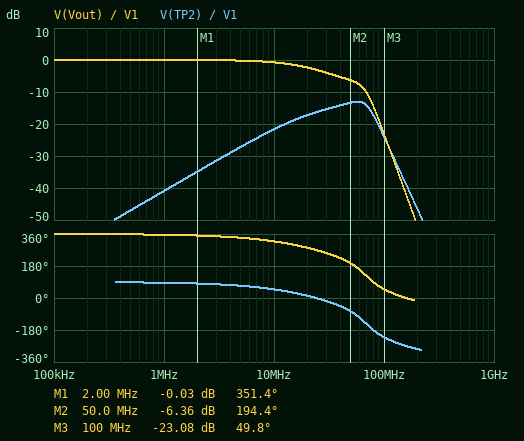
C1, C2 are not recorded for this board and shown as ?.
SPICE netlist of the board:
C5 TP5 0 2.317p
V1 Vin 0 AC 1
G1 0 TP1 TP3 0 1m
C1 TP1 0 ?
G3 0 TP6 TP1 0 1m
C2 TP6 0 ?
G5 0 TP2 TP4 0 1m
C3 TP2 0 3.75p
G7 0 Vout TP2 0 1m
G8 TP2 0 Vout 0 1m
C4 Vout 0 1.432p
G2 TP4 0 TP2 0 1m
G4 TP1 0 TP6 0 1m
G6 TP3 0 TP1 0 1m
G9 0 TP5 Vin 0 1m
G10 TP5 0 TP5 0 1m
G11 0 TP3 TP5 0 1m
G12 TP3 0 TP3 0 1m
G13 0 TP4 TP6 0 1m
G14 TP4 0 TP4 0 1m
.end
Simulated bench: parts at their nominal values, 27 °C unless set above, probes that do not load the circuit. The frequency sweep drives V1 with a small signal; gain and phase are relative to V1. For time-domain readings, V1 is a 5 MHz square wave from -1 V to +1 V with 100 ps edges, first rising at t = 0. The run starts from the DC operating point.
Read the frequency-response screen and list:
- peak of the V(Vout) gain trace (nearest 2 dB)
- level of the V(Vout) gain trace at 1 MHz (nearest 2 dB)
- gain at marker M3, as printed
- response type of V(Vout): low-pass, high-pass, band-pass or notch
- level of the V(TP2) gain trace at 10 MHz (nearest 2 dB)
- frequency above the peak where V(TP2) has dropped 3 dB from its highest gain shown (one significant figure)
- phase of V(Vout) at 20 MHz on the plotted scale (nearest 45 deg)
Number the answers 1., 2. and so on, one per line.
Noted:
1. 0 dB
2. 0 dB
3. -23.08 dB
4. low-pass
5. -22 dB
6. 80 MHz
7. 270 deg
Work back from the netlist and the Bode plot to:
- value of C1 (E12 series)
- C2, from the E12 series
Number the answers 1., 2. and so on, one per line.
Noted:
1. 1 pF
2. 8.2 pF
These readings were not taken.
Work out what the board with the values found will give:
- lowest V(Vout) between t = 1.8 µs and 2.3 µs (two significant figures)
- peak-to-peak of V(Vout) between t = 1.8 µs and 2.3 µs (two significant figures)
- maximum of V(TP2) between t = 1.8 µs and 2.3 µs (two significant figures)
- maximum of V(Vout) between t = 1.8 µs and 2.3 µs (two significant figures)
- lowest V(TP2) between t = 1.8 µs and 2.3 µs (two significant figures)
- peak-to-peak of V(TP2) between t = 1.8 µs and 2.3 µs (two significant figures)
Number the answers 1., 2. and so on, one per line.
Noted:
1. -1.0 V
2. 2.0 V
3. 280 mV
4. 1.0 V
5. -280 mV
6. 560 mV
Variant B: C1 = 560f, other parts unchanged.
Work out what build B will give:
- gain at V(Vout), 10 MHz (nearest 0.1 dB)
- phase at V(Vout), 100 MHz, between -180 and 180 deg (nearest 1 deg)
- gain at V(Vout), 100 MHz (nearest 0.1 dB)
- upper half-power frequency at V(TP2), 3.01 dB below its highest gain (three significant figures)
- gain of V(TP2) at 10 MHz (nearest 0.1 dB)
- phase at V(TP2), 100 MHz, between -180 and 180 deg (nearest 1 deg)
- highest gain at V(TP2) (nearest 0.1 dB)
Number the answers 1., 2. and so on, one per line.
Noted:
1. -0.8 dB
2. 64 deg
3. -22.4 dB
4. 77.0 MHz
5. -21.8 dB
6. 154 deg
7. -13.1 dB
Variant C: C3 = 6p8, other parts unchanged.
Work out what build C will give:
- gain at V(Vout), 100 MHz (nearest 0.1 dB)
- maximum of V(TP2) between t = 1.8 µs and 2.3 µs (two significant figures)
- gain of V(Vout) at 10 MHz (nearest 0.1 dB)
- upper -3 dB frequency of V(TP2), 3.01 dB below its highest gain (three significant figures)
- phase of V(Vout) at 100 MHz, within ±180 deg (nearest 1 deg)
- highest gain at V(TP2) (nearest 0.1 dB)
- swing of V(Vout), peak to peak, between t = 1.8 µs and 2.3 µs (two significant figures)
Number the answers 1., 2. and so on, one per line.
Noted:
1. -29.4 dB
2. 290 mV
3. -0.6 dB
4. 57.8 MHz
5. 29 deg
6. -9.9 dB
7. 2.1 V
